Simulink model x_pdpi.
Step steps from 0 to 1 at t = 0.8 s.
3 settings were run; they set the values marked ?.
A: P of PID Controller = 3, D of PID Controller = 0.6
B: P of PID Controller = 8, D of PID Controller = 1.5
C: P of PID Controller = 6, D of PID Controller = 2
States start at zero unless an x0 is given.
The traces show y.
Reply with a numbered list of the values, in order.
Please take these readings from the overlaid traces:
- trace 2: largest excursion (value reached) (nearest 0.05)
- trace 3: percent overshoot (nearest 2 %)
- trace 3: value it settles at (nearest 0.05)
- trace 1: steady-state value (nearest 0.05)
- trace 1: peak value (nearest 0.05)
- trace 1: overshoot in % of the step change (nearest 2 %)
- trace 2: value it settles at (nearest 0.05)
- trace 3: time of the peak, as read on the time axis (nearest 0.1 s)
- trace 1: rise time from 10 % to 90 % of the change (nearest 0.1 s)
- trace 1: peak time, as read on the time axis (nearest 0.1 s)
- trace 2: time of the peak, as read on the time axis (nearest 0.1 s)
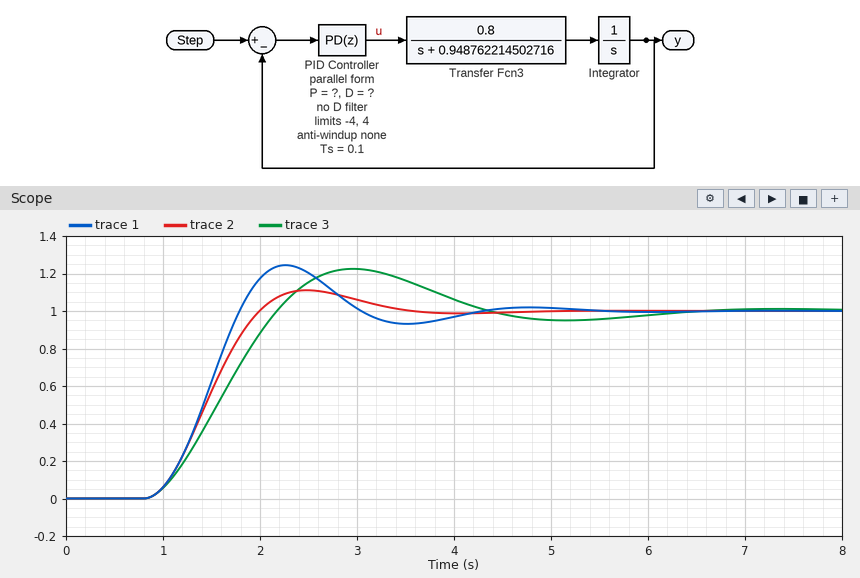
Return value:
1. 1.10
2. 22 %
3. 1.00
4. 1.00
5. 1.25
6. 24 %
7. 1.00
8. 3.0 s
9. 0.6 s
10. 2.3 s
11. 2.5 s
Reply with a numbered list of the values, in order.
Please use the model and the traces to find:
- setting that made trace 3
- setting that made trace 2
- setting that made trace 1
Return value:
1. A
2. C
3. B
